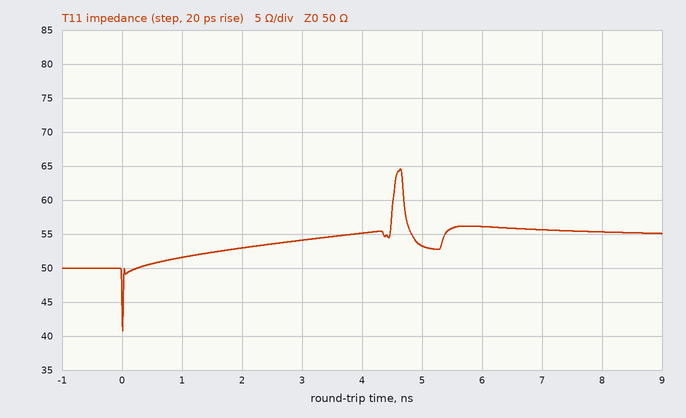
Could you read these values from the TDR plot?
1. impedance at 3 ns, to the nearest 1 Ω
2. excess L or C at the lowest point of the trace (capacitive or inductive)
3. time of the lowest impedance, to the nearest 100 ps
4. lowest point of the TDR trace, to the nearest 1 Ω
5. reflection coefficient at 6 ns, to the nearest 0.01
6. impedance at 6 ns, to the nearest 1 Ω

54 Ω
capacitive
0.0 ns
41 Ω
+0.06
56 Ω
